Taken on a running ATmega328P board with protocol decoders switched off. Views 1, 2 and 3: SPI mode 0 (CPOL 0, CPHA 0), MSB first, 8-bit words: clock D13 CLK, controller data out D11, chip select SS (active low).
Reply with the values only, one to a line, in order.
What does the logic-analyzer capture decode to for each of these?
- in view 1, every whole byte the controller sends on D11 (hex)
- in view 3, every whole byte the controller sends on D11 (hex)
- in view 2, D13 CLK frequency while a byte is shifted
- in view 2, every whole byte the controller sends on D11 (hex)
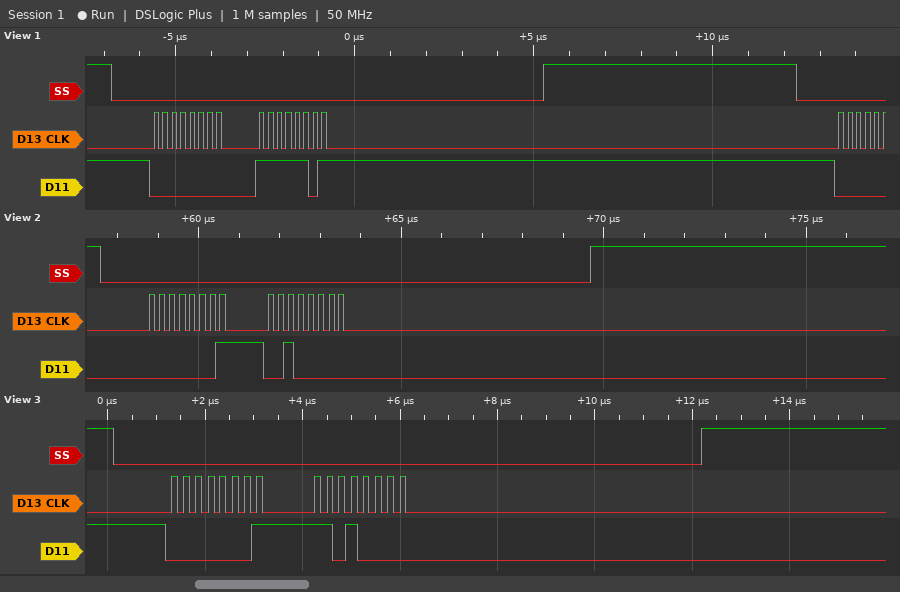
00 FD
01 D0
4 MHz
01 20
